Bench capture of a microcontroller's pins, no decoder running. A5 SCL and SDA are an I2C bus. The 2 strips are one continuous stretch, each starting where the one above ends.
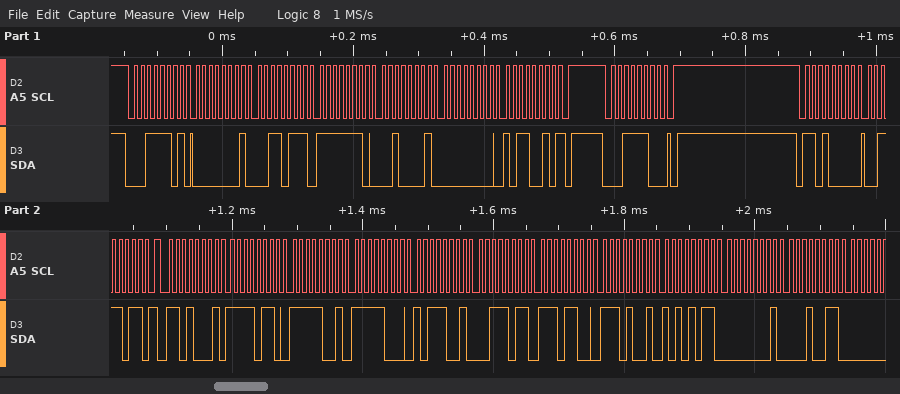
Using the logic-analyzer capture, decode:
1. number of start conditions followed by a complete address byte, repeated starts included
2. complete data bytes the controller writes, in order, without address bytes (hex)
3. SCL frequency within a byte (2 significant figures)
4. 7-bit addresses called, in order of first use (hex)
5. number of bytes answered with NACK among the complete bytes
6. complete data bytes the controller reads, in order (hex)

4
3B
100 kHz
0x1E 0x68
1
01 37 FE 21 00 B2 F6 F9 F8 B9 3B EC E9 AB 01 13
